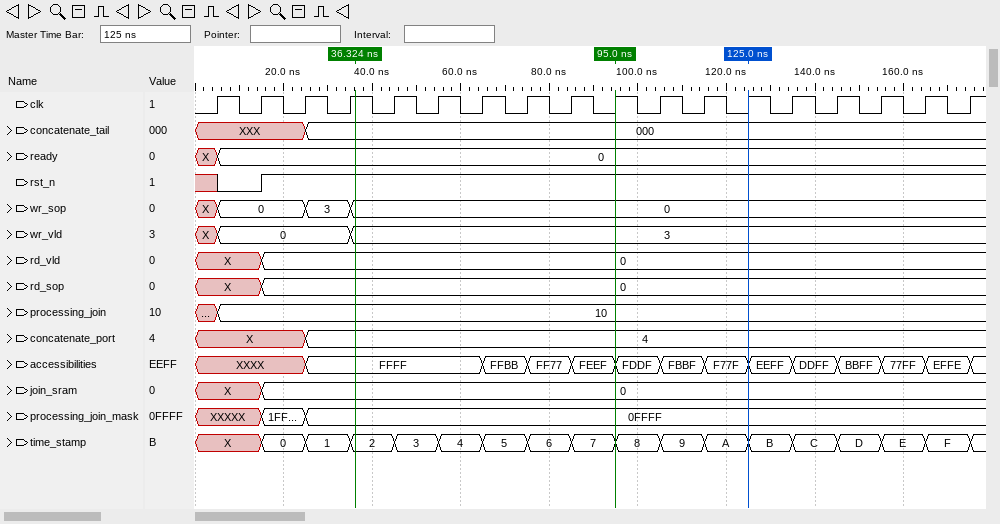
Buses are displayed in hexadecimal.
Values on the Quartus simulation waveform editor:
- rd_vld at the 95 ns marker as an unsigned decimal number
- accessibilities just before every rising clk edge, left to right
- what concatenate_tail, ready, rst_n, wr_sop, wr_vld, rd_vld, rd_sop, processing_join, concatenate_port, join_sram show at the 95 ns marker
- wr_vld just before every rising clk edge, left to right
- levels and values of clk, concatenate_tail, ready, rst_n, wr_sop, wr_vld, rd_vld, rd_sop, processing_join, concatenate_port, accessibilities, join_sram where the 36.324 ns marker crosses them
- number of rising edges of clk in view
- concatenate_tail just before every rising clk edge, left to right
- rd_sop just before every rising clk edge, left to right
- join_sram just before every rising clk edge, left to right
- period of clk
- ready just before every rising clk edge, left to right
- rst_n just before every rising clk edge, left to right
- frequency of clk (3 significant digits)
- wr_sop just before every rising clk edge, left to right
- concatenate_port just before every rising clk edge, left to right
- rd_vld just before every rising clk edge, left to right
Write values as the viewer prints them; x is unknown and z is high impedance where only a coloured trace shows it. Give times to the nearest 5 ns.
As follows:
0
XXXX, XXXX, XXXX, FFFF, FFFF, FFFF, FFFF, FFBB, FF77, FEEF, FDDF, FBBF, F77F, EEFF, DDFF, BBFF, 77FF, EFFE
concatenate_tail=000, ready=0, rst_n=1, wr_sop=0, wr_vld=3, rd_vld=0, rd_sop=0, processing_join=10, concatenate_port=4, join_sram=0
X, 0, 0, 0, 3, 3, 3, 3, 3, 3, 3, 3, 3, 3, 3, 3, 3, 3
clk=1, concatenate_tail=000, ready=0, rst_n=1, wr_sop=0, wr_vld=3, rd_vld=0, rd_sop=0, processing_join=10, concatenate_port=4, accessibilities=FFFF, join_sram=0
18
XXX, XXX, XXX, 000, 000, 000, 000, 000, 000, 000, 000, 000, 000, 000, 000, 000, 000, 000
X, X, 0, 0, 0, 0, 0, 0, 0, 0, 0, 0, 0, 0, 0, 0, 0, 0
X, X, 0, 0, 0, 0, 0, 0, 0, 0, 0, 0, 0, 0, 0, 0, 0, 0
10 ns
X, 0, 0, 0, 0, 0, 0, 0, 0, 0, 0, 0, 0, 0, 0, 0, 0, 0
x 0 1 1 1 1 1 1 1 1 1 1 1 1 1 1 1 1
100 MHz
X, 0, 0, 3, 0, 0, 0, 0, 0, 0, 0, 0, 0, 0, 0, 0, 0, 0
X, X, X, 4, 4, 4, 4, 4, 4, 4, 4, 4, 4, 4, 4, 4, 4, 4
X, X, 0, 0, 0, 0, 0, 0, 0, 0, 0, 0, 0, 0, 0, 0, 0, 0
